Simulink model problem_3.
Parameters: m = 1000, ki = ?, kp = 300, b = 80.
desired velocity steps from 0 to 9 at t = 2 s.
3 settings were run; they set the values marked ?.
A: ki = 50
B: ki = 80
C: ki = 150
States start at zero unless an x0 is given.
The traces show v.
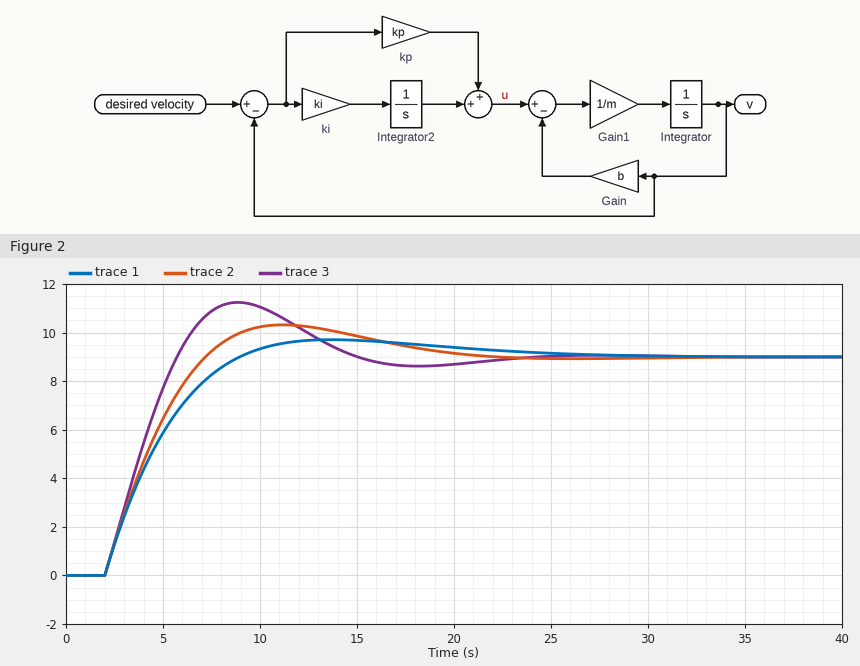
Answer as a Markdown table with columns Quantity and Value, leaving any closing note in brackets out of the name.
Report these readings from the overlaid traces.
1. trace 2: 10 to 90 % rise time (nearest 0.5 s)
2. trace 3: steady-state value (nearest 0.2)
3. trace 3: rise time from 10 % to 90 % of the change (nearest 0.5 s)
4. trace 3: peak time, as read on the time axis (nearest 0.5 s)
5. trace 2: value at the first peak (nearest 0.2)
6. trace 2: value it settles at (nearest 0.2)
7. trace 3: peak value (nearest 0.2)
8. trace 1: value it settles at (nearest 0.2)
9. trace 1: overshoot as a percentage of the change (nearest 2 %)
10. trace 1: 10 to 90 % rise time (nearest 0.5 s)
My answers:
| Quantity | Value |
|---|---|
| trace 2: 10 to 90 % rise time | 4.0 s |
| trace 3: steady-state value | 9.0 |
| trace 3: rise time from 10 % to 90 % of the change | 3.0 s |
| trace 3: peak time, as read on the time axis | 9.0 s |
| trace 2: value at the first peak | 10.4 |
| trace 2: value it settles at | 9.0 |
| trace 3: peak value | 11.2 |
| trace 1: value it settles at | 9.0 |
| trace 1: overshoot as a percentage of the change | 8 % |
| trace 1: 10 to 90 % rise time | 5.0 s |
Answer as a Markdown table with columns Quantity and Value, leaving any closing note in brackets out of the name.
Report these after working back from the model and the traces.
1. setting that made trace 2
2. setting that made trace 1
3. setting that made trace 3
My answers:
| Quantity | Value |
|---|---|
| setting that made trace 2 | B |
| setting that made trace 1 | A |
| setting that made trace 3 | C |
